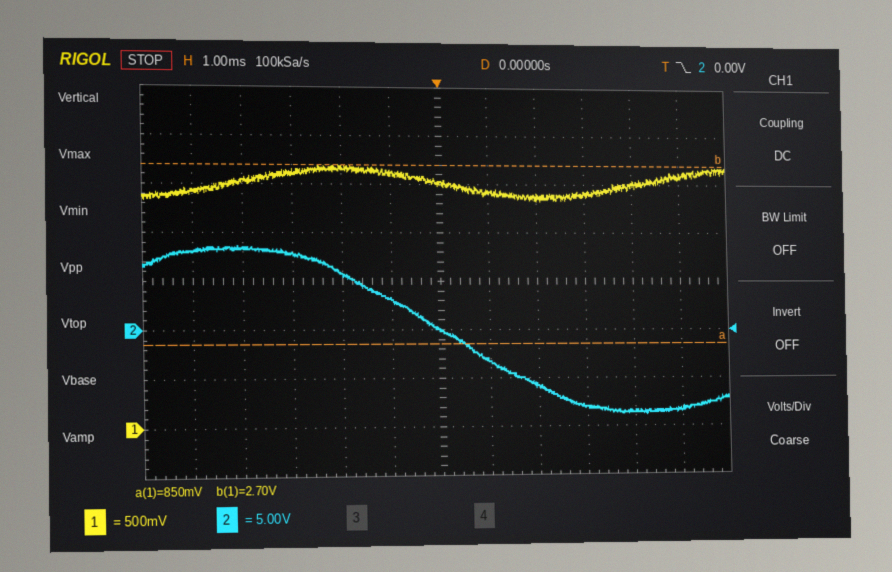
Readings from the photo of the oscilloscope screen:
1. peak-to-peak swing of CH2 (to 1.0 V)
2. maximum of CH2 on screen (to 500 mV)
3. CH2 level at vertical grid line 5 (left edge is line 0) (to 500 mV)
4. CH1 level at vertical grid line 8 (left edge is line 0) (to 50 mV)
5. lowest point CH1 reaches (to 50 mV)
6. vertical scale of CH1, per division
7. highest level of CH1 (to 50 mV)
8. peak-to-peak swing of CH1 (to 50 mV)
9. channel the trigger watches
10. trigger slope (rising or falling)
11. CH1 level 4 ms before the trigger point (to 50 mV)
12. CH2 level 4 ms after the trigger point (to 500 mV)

17.0 V
8.5 V
3.0 V
2.35 V
2.35 V
500 mV
2.70 V
350 mV
CH2
falling
2.55 V
-8.5 V
